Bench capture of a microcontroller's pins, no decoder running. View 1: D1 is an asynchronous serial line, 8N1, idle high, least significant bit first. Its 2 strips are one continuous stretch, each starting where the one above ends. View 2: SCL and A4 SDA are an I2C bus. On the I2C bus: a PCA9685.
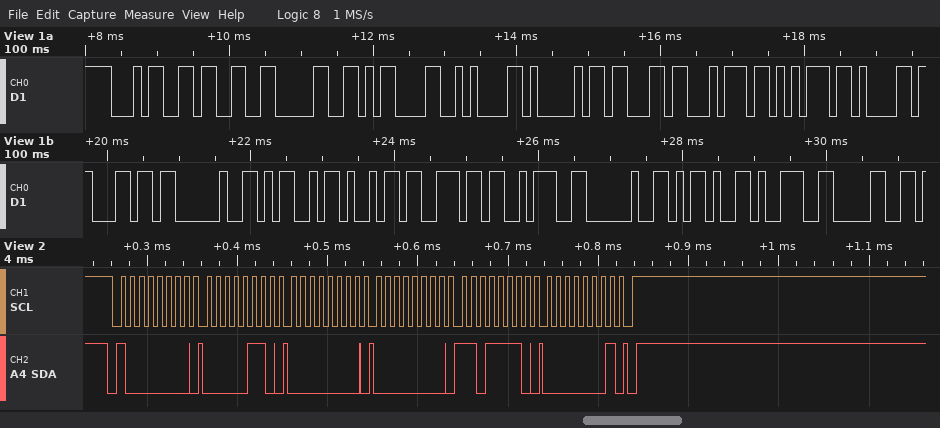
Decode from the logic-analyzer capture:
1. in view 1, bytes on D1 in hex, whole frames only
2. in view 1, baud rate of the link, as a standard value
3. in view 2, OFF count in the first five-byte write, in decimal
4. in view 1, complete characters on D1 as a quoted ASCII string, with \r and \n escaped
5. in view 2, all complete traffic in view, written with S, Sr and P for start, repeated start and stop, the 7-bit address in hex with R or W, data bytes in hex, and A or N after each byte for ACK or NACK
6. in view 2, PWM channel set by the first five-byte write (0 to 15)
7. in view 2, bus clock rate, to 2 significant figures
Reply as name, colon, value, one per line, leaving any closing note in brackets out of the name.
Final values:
in view 1, bytes on D1 in hex, whole frames only: 0x34 0x33 0x30 0x0D 0x0A 0x41 0x63 0x74 0x75 0x61 0x6C 0x20 0x4D 0x69 0x6E 0x3A 0x20 0x2D 0x39 0x30
in view 1, baud rate of the link, as a standard value: 9600 baud
in view 2, OFF count in the first five-byte write, in decimal: 478
in view 1, complete characters on D1 as a quoted ASCII string, with \r and \n escaped: "430\r\nActual Min: -90"
in view 2, all complete traffic in view, written with S, Sr and P for start, repeated start and stop, the 7-bit address in hex with R or W, data bytes in hex, and A or N after each byte for ACK or NACK: S 40W A 06 A 00 A 00 A DE A 01 A P
in view 2, PWM channel set by the first five-byte write: 0
in view 2, bus clock rate, to 2 significant figures: 100 kHz
